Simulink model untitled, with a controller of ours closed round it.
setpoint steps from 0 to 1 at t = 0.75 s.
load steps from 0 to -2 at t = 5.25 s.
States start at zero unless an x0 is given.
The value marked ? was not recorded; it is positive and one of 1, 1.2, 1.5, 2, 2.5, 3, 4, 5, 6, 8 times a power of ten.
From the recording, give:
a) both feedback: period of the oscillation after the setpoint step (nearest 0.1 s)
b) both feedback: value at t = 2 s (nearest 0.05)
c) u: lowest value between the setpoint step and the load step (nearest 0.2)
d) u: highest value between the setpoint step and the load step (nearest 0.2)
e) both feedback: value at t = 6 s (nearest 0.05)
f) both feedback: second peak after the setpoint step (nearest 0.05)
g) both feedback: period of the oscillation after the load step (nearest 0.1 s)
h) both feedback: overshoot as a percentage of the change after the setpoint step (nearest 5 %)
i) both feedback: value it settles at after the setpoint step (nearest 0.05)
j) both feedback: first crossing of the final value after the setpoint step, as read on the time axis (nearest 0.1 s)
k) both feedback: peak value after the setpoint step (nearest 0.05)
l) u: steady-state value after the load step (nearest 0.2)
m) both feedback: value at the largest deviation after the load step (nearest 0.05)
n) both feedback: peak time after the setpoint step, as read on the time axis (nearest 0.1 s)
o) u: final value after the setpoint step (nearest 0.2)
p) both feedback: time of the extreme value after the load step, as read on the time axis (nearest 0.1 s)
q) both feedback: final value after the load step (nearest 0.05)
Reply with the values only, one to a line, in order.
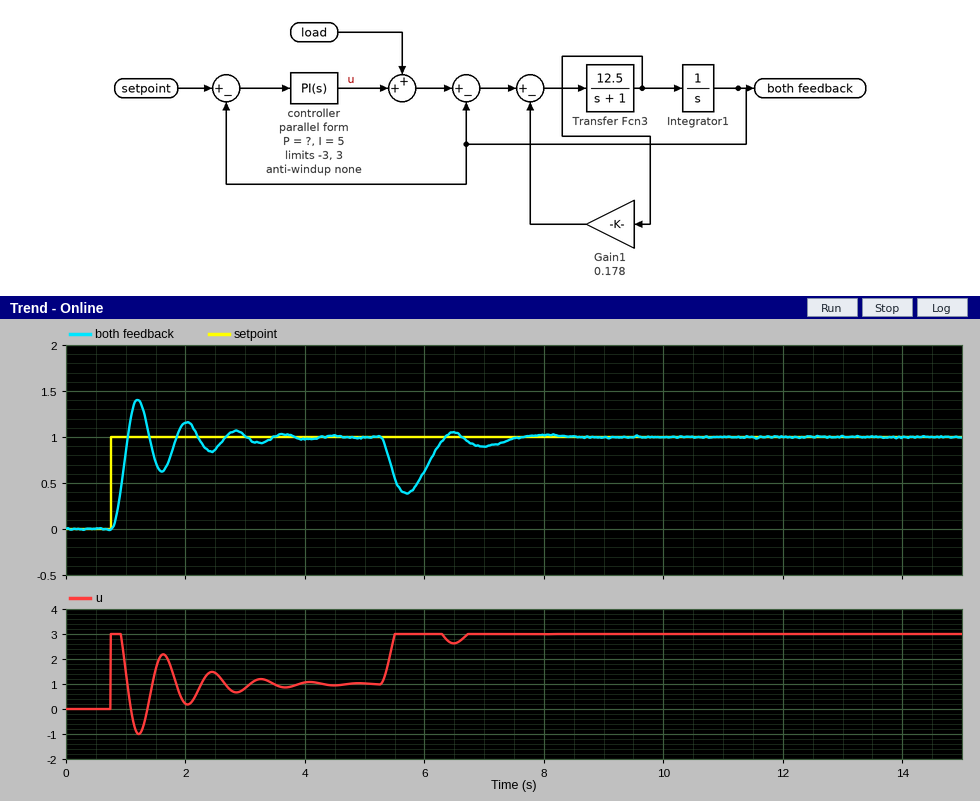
0.8 s
1.15
-1.0
3.0
0.65
1.15
1.3 s
40 %
1.00
1.0 s
1.40
3.0
0.40
1.2 s
1.0
5.7 s
1.00
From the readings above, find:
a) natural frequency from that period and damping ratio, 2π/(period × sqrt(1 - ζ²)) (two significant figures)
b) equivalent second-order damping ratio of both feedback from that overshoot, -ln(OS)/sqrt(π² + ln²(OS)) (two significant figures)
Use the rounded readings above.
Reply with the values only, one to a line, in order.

8.2 rad/s
0.28
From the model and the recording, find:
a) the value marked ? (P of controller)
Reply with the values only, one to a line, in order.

4
